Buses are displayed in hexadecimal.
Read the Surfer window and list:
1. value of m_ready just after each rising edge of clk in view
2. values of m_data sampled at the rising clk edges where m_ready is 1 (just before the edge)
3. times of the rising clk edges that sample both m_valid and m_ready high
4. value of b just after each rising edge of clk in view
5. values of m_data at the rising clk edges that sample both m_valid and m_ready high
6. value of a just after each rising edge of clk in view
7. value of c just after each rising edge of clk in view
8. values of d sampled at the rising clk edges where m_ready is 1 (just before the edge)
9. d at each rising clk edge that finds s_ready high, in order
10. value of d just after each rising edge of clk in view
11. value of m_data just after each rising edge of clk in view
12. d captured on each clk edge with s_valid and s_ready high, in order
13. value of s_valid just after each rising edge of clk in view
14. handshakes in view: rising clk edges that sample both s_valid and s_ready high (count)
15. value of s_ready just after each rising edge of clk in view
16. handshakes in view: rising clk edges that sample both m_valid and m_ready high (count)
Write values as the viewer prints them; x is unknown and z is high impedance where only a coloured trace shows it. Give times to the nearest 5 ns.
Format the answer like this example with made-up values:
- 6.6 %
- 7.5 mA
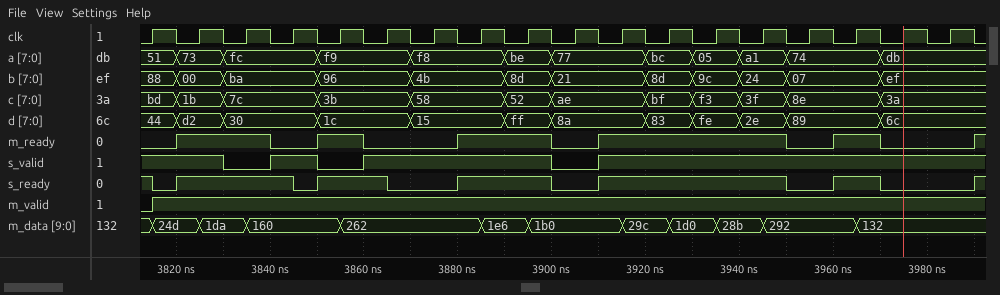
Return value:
- 0 1 1 0 1 0 0 1 1 0 1 1 1 1 0 1 0 0
- 24d, 1da, 160, 262, 1e6, 1b0, 29c, 1d0, 28b, 292
- 3825 ns, 3835 ns, 3855 ns, 3885 ns, 3895 ns, 3915 ns, 3925 ns, 3935 ns, 3945 ns, 3965 ns
- 88, 00, ba, ba, 96, 96, 4b, 4b, 8d, 21, 21, 8d, 9c, 24, 07, 07, ef, ef
- 24d, 1da, 160, 262, 1e6, 1b0, 29c, 1d0, 28b, 292
- 51, 73, fc, fc, f9, f9, f8, f8, be, 77, 77, bc, 05, a1, 74, 74, db, db
- bd, 1b, 7c, 7c, 3b, 3b, 58, 58, 52, ae, ae, bf, f3, 3f, 8e, 8e, 3a, 3a
- d2, 30, 1c, 15, ff, 8a, 83, fe, 2e, 89
- 44, d2, 30, 30, 1c, 1c, 15, ff, 8a, 83, fe, 2e, 89
- 44, d2, 30, 30, 1c, 1c, 15, 15, ff, 8a, 8a, 83, fe, 2e, 89, 89, 6c, 6c
- 24d, 1da, 160, 160, 262, 262, 262, 1e6, 1b0, 1b0, 29c, 1d0, 28b, 292, 292, 132, 132, 132
- 44, d2, 30, 1c, 15, ff, 8a, 83, fe, 2e, 89
- 1 1 0 1 0 1 1 1 1 0 1 1 1 1 1 1 1 1
- 11
- 0 1 1 0 1 0 0 1 1 0 1 1 1 1 0 1 0 0
- 10
